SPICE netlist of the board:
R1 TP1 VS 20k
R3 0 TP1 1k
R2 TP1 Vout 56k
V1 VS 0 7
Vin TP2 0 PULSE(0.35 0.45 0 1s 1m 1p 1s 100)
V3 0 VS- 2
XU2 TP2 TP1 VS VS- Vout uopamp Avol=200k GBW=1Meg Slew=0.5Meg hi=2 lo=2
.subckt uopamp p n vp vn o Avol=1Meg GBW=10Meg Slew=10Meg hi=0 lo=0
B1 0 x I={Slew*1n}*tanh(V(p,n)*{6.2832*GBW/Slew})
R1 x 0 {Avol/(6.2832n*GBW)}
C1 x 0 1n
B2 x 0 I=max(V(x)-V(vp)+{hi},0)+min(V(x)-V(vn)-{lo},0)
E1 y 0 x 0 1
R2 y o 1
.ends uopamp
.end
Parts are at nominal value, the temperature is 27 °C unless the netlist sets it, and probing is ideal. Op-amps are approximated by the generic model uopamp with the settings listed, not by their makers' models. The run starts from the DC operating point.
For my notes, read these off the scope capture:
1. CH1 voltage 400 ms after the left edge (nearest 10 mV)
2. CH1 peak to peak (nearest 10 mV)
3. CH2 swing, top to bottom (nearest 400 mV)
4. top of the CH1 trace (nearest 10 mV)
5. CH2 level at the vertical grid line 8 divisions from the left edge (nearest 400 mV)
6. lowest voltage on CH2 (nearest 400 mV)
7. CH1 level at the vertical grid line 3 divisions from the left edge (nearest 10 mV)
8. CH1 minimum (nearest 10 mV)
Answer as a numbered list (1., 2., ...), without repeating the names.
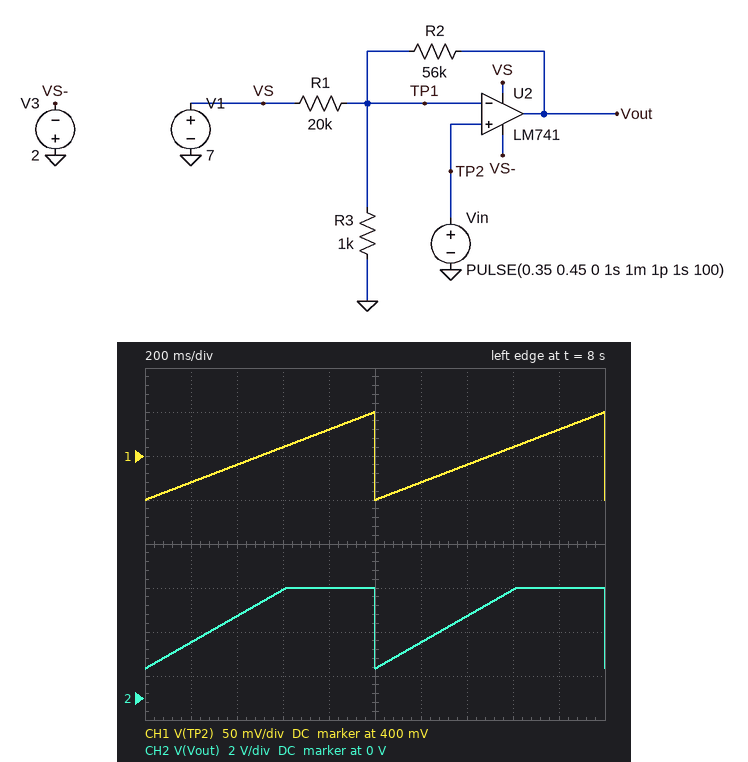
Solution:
1. 390 mV
2. 100 mV
3. 3.6 V
4. 450 mV
5. 4.8 V
6. 1.2 V
7. 410 mV
8. 350 mV
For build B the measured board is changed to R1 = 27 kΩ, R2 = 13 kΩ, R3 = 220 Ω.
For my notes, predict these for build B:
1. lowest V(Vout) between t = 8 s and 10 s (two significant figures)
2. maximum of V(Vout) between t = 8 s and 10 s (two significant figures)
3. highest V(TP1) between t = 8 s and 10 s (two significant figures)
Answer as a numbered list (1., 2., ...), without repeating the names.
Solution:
1. 5.0 V
2. 5.0 V
3. 140 mV
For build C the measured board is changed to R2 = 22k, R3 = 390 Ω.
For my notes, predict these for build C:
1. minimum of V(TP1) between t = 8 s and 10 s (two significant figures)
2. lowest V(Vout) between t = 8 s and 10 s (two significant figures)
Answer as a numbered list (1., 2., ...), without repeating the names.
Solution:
1. 220 mV
2. 5.0 V
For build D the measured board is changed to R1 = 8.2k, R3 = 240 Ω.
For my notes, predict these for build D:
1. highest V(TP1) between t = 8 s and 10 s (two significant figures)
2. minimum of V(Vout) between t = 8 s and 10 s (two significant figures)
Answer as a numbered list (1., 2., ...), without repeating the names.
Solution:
1. 220 mV
2. 5.0 V
